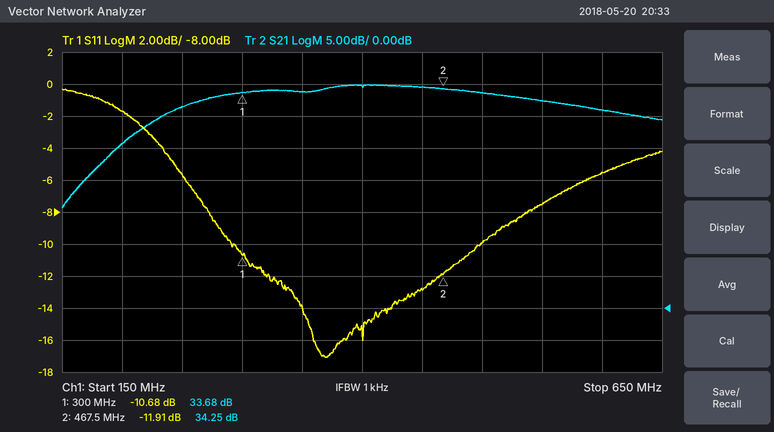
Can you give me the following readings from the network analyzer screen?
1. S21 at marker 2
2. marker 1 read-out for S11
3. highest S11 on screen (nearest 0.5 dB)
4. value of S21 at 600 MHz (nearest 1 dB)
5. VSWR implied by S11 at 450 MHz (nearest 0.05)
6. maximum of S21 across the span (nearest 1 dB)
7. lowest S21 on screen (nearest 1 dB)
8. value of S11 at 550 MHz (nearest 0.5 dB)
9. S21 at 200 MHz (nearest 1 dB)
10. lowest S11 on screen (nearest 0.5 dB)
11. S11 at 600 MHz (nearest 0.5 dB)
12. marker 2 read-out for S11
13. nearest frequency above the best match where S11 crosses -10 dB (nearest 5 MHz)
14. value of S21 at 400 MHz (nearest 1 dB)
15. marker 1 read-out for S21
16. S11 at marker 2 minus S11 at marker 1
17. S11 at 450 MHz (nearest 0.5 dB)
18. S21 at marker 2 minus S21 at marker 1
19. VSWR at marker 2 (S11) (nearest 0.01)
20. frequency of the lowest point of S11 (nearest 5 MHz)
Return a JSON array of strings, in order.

["34.25 dB", "-10.68 dB", "-0.5 dB", "31 dB", "1.60", "35 dB", "16 dB", "-7.5 dB", "26 dB", "-17.0 dB", "-5.5 dB", "-11.91 dB", "500 MHz", "35 dB", "33.68 dB", "-1.23 dB", "-13.0 dB", "0.57 dB", "1.68", "370 MHz"]
